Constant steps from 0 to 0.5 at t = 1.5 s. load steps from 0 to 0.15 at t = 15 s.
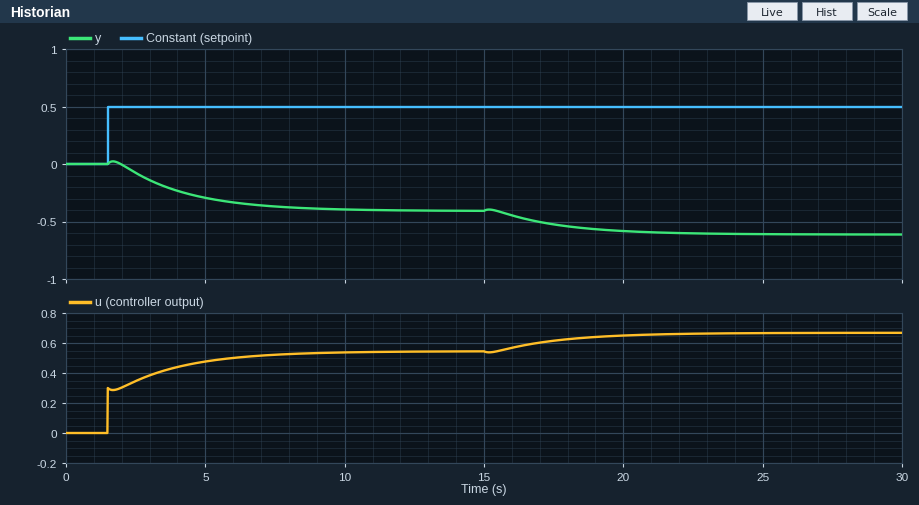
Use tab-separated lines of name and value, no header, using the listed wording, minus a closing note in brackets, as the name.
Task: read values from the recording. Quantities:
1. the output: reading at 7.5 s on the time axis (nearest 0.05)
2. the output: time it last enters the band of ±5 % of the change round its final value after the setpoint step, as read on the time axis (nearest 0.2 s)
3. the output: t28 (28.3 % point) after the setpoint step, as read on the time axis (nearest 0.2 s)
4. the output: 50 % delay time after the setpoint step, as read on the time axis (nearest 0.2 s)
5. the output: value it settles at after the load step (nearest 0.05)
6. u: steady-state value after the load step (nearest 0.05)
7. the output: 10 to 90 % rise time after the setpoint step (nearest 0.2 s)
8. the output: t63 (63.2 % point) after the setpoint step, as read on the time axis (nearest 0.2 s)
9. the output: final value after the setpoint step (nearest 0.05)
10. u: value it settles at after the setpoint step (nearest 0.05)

the output: reading at 7.5 s on the time axis	-0.35
the output: time it last enters the band of ±5 % of the change round its final value after the setpoint step, as read on the time axis	9.0 s
the output: t28 (28.3 % point) after the setpoint step, as read on the time axis	2.8 s
the output: 50 % delay time after the setpoint step, as read on the time axis	3.6 s
the output: value it settles at after the load step	-0.60
u: steady-state value after the load step	0.65
the output: 10 to 90 % rise time after the setpoint step	5.2 s
the output: t63 (63.2 % point) after the setpoint step, as read on the time axis	4.4 s
the output: final value after the setpoint step	-0.40
u: value it settles at after the setpoint step	0.55
